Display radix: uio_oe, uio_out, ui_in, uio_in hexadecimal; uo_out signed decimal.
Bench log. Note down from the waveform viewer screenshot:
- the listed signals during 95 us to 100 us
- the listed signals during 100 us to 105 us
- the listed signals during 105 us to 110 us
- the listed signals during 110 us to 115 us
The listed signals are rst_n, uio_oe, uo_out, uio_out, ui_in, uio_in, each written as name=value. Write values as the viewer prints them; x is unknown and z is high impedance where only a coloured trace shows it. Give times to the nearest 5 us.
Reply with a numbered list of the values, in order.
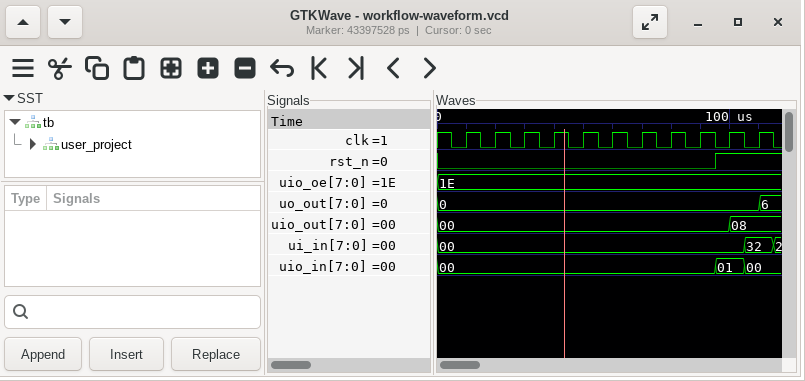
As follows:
1. rst_n=1, uio_oe=1E, uo_out=0, uio_out=00, ui_in=00, uio_in=01
2. rst_n=1, uio_oe=1E, uo_out=0, uio_out=08, ui_in=00, uio_in=01
3. rst_n=1, uio_oe=1E, uo_out=0, uio_out=08, ui_in=32, uio_in=00
4. rst_n=1, uio_oe=1E, uo_out=6, uio_out=08, ui_in=32, uio_in=00
